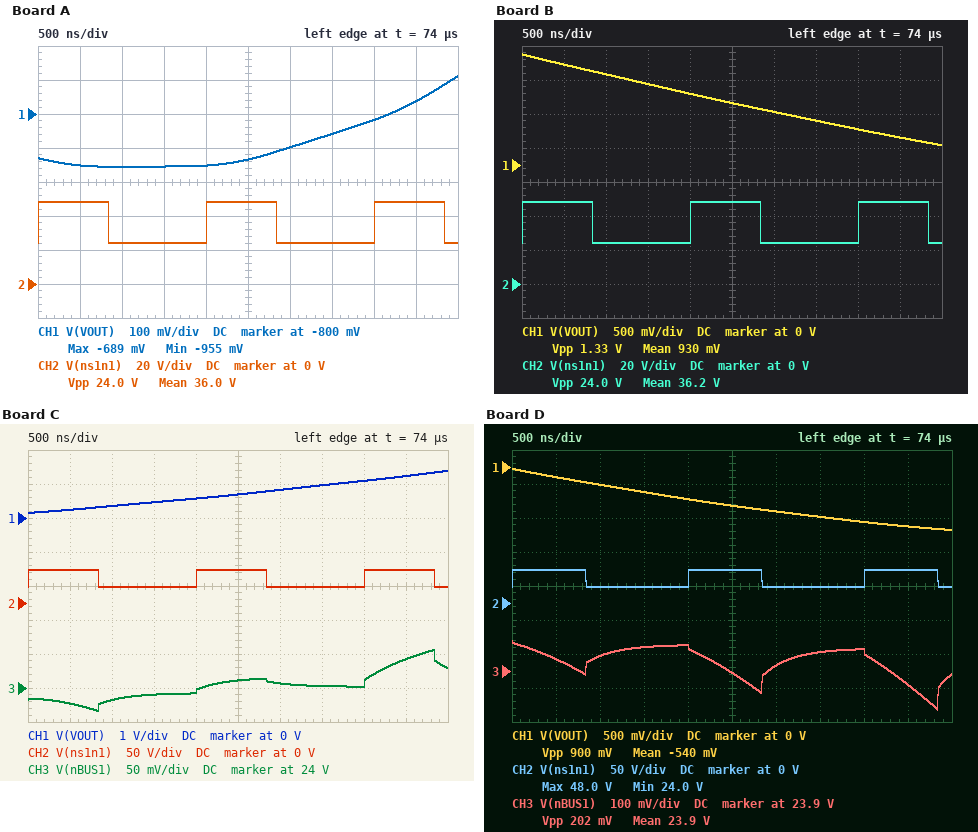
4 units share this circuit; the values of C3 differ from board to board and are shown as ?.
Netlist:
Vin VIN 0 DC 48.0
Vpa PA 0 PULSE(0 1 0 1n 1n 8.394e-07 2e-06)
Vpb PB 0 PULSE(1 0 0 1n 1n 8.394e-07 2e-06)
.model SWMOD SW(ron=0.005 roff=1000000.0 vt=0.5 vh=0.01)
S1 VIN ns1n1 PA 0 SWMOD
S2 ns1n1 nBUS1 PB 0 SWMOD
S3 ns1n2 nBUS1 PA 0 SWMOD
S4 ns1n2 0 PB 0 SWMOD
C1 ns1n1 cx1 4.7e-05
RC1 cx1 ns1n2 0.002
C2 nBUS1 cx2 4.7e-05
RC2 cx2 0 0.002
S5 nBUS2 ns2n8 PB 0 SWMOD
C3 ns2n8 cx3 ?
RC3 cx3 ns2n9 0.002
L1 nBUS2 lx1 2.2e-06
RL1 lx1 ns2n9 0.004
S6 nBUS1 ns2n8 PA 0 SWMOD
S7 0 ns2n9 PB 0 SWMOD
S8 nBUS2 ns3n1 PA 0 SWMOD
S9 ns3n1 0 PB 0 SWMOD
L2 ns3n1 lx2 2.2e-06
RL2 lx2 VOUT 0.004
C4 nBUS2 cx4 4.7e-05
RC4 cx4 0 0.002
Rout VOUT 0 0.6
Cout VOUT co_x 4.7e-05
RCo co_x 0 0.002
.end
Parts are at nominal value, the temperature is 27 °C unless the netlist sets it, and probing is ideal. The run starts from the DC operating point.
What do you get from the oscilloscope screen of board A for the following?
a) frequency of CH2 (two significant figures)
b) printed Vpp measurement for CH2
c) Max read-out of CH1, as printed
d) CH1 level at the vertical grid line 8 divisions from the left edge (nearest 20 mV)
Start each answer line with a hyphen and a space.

- 500 kHz
- 24.0 V
- -689 mV
- -820 mV
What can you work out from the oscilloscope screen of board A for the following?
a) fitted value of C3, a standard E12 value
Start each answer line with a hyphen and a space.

- 39 µF
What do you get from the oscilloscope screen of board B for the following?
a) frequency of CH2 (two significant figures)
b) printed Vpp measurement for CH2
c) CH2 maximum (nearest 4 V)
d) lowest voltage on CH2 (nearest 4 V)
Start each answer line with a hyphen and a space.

- 500 kHz
- 24.0 V
- 48 V
- 24 V
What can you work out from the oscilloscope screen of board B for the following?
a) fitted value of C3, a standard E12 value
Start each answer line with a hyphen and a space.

- 100 µF
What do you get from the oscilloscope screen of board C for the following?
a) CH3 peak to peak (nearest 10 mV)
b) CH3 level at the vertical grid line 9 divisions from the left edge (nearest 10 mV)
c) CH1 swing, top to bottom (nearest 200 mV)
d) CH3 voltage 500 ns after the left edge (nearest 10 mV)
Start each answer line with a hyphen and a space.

- 90 mV
- 24.04 V
- 1.2 V
- 23.98 V
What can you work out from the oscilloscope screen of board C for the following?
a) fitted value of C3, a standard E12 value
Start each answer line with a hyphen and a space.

- 18 µF
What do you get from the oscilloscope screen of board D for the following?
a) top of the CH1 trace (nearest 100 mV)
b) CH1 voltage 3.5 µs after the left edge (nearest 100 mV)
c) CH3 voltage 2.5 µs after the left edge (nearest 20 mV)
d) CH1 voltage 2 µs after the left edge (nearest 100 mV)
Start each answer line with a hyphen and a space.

- 0 V
- -700 mV
- 23.90 V
- -500 mV
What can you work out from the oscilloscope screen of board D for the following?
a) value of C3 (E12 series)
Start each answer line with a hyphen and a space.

- 68 µF
